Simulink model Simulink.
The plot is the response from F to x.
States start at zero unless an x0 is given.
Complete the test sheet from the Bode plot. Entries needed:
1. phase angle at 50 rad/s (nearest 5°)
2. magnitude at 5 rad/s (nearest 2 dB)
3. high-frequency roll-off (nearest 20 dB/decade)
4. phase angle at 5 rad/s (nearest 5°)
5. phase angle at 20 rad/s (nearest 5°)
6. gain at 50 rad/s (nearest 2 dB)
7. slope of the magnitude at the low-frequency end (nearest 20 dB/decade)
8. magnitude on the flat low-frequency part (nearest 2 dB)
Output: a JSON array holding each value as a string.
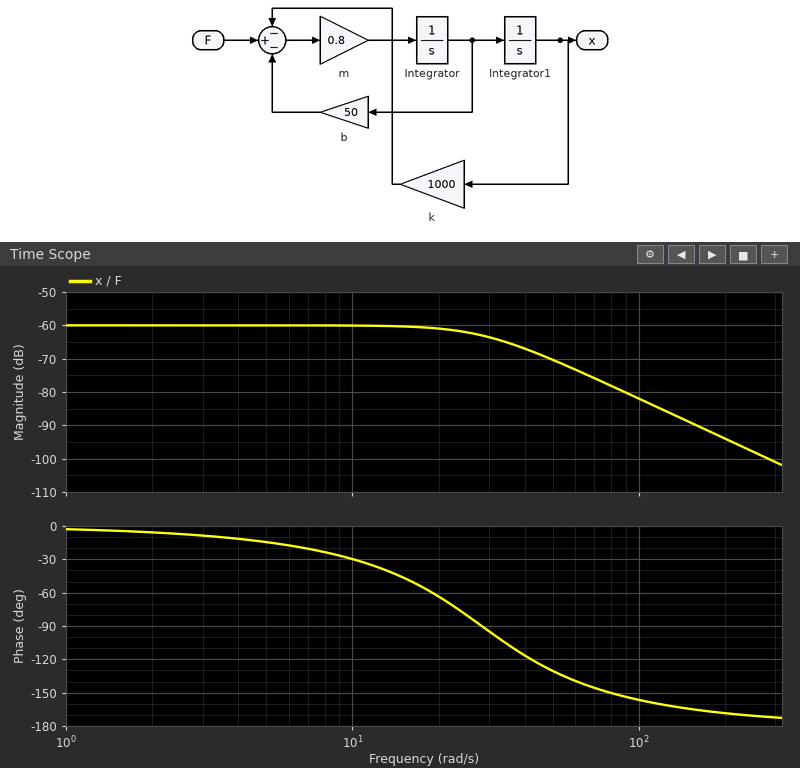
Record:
["-130°", "-60 dB", "-40 dB/decade", "-15°", "-65°", "-70 dB", "0 dB/decade", "-60 dB"]
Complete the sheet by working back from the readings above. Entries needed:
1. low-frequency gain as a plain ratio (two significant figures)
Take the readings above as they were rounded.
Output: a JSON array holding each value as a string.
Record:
["0.0010"]
